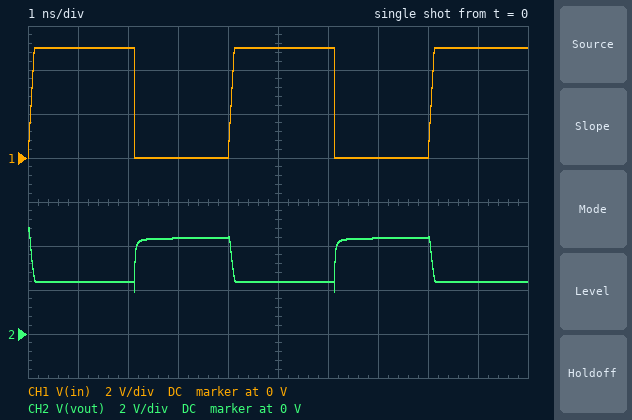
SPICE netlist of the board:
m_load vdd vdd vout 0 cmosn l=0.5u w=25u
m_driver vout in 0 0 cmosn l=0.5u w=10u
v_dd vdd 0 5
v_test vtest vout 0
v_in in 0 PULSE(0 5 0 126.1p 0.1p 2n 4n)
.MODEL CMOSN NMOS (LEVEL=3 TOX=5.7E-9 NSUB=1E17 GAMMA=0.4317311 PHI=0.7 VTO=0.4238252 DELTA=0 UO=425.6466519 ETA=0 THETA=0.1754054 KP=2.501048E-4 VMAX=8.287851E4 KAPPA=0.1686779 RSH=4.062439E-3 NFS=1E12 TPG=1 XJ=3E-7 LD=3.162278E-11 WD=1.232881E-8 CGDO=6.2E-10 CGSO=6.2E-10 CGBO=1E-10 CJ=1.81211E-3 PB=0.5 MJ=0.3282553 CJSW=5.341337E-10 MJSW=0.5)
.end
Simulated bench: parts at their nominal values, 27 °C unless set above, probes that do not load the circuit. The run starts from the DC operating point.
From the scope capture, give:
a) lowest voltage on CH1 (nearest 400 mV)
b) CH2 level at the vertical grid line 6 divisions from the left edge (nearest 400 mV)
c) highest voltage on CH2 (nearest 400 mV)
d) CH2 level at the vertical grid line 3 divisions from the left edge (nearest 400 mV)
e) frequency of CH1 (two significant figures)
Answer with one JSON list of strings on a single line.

["0 V", "2.4 V", "4.8 V", "4.4 V", "250 MHz"]
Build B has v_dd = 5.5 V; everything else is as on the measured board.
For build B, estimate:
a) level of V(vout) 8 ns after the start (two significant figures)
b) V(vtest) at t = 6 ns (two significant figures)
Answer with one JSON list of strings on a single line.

["4.9 V", "2.8 V"]
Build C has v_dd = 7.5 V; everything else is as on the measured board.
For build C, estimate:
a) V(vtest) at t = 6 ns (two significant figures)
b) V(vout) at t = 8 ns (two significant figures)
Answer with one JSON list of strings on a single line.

["4.6 V", "6.8 V"]
